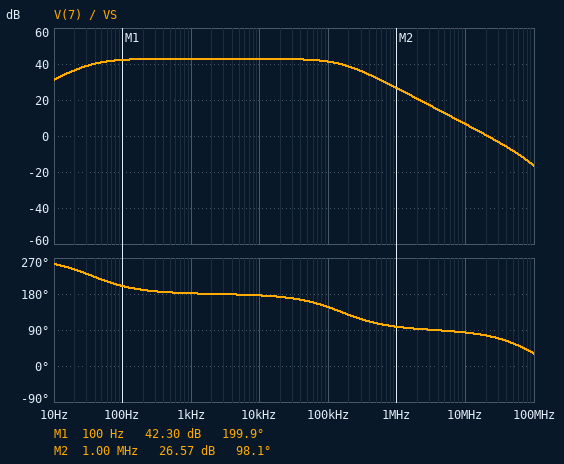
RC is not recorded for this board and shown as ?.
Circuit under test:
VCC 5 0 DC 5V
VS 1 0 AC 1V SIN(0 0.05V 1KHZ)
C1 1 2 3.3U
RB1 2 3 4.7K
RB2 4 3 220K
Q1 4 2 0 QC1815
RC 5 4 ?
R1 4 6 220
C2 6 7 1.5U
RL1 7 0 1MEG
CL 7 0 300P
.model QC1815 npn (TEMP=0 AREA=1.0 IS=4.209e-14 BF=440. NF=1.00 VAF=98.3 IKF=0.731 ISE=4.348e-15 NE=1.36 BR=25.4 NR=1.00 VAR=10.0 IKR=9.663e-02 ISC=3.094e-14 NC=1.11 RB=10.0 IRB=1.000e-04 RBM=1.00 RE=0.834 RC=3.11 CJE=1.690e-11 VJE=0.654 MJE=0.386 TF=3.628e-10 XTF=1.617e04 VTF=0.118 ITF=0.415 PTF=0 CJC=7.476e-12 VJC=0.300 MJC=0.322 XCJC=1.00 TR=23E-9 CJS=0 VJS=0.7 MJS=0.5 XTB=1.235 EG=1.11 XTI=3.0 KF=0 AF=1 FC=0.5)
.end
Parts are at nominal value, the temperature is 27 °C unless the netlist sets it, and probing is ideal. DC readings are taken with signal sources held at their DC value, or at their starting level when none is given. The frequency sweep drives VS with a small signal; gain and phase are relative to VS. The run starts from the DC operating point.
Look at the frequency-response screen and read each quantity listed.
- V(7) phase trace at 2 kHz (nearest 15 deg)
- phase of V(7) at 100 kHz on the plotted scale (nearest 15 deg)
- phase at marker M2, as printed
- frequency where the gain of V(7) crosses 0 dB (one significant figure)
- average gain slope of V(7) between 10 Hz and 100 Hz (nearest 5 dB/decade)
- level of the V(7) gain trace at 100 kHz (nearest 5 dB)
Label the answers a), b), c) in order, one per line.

a) 180 deg
b) 150 deg
c) 98.1 deg
d) 20 MHz
e) 10 dB/decade
f) 40 dB
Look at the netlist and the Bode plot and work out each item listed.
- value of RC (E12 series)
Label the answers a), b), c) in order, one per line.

a) 3.3 kΩ
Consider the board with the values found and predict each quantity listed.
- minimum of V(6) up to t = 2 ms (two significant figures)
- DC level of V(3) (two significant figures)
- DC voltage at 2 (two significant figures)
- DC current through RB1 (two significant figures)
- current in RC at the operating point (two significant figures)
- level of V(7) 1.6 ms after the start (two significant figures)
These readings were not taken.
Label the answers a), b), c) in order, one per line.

a) 19 mV
b) 690 mV
c) 670 mV
d) 3.2 µA
e) 1.1 mA
f) 3.2 V
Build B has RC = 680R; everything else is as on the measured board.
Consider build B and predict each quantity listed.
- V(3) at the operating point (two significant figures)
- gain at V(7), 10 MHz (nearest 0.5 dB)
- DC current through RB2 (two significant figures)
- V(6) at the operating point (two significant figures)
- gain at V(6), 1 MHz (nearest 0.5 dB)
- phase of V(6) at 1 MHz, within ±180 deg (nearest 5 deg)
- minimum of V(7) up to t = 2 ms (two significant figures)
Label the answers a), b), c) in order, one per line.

a) 740 mV
b) 13.5 dB
c) 9.3 µA
d) 2.8 V
e) 32.5 dB
f) 120 deg
g) -2.7 V
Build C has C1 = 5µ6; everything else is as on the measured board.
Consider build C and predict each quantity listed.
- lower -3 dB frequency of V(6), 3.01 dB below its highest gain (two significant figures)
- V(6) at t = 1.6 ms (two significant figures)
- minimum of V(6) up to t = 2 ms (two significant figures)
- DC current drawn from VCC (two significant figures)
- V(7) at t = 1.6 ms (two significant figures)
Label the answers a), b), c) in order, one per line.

a) 21 Hz
b) 4.5 V
c) 18 mV
d) 1.1 mA
e) 3.1 V
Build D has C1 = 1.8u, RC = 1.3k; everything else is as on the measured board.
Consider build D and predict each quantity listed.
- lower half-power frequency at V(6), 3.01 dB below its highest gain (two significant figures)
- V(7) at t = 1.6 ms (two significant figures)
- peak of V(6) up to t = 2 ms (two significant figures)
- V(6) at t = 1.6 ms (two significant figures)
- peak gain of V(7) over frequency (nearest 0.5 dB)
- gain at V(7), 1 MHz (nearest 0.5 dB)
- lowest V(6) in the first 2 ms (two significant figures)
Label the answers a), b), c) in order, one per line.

a) 65 Hz
b) 2.6 V
c) 4.9 V
d) 4.7 V
e) 40.5 dB
f) 31.0 dB
g) 41 mV
